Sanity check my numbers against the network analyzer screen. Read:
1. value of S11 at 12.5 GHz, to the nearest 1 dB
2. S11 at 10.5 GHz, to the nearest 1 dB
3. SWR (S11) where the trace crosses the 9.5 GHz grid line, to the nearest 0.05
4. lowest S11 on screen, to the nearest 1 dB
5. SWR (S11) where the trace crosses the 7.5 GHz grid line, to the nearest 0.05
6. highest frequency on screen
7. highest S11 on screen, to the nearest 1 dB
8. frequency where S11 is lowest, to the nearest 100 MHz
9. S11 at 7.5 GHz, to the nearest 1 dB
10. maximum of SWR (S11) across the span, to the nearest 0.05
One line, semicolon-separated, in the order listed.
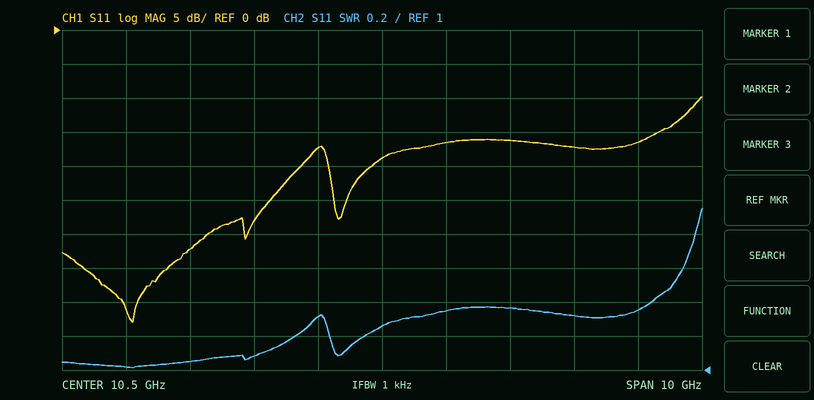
-16 dB; -19 dB; 1.30; -43 dB; 1.05; 15.5 GHz; -10 dB; 6.6 GHz; -32 dB; 1.95
